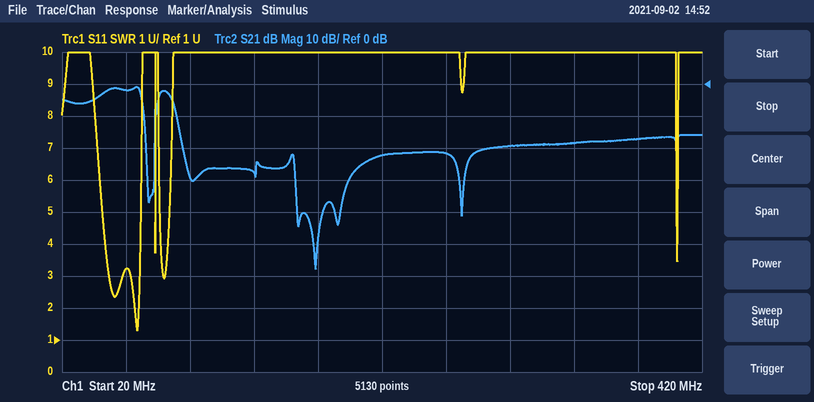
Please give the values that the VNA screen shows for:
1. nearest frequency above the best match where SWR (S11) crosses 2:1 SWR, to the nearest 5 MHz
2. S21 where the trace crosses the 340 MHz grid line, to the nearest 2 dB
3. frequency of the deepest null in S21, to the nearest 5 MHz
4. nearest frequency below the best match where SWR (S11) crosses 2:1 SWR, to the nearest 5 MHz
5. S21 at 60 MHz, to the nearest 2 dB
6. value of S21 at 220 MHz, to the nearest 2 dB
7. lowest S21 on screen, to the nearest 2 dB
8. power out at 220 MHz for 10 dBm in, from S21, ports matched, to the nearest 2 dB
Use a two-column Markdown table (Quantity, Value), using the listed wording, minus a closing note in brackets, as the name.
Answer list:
| Quantity | Value |
|---|---|
| nearest frequency above the best match where SWR (S11) crosses 2:1 SWR, to the nearest 5 MHz | 70 MHz |
| S21 where the trace crosses the 340 MHz grid line, to the nearest 2 dB | -18 dB |
| frequency of the deepest null in S21, to the nearest 5 MHz | 180 MHz |
| nearest frequency below the best match where SWR (S11) crosses 2:1 SWR, to the nearest 5 MHz | 65 MHz |
| S21 at 60 MHz, to the nearest 2 dB | -2 dB |
| value of S21 at 220 MHz, to the nearest 2 dB | -22 dB |
| lowest S21 on screen, to the nearest 2 dB | -58 dB |
| power out at 220 MHz for 10 dBm in, from S21, ports matched, to the nearest 2 dB | -12 dBm |
